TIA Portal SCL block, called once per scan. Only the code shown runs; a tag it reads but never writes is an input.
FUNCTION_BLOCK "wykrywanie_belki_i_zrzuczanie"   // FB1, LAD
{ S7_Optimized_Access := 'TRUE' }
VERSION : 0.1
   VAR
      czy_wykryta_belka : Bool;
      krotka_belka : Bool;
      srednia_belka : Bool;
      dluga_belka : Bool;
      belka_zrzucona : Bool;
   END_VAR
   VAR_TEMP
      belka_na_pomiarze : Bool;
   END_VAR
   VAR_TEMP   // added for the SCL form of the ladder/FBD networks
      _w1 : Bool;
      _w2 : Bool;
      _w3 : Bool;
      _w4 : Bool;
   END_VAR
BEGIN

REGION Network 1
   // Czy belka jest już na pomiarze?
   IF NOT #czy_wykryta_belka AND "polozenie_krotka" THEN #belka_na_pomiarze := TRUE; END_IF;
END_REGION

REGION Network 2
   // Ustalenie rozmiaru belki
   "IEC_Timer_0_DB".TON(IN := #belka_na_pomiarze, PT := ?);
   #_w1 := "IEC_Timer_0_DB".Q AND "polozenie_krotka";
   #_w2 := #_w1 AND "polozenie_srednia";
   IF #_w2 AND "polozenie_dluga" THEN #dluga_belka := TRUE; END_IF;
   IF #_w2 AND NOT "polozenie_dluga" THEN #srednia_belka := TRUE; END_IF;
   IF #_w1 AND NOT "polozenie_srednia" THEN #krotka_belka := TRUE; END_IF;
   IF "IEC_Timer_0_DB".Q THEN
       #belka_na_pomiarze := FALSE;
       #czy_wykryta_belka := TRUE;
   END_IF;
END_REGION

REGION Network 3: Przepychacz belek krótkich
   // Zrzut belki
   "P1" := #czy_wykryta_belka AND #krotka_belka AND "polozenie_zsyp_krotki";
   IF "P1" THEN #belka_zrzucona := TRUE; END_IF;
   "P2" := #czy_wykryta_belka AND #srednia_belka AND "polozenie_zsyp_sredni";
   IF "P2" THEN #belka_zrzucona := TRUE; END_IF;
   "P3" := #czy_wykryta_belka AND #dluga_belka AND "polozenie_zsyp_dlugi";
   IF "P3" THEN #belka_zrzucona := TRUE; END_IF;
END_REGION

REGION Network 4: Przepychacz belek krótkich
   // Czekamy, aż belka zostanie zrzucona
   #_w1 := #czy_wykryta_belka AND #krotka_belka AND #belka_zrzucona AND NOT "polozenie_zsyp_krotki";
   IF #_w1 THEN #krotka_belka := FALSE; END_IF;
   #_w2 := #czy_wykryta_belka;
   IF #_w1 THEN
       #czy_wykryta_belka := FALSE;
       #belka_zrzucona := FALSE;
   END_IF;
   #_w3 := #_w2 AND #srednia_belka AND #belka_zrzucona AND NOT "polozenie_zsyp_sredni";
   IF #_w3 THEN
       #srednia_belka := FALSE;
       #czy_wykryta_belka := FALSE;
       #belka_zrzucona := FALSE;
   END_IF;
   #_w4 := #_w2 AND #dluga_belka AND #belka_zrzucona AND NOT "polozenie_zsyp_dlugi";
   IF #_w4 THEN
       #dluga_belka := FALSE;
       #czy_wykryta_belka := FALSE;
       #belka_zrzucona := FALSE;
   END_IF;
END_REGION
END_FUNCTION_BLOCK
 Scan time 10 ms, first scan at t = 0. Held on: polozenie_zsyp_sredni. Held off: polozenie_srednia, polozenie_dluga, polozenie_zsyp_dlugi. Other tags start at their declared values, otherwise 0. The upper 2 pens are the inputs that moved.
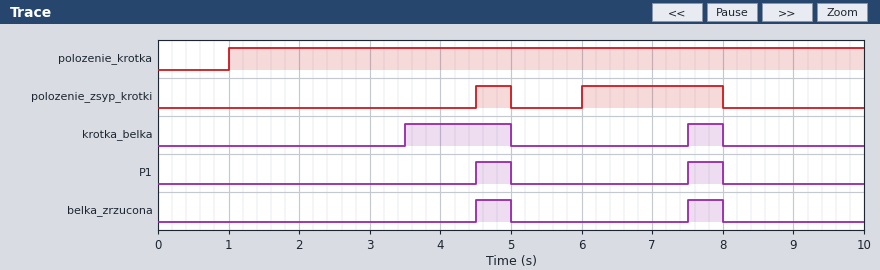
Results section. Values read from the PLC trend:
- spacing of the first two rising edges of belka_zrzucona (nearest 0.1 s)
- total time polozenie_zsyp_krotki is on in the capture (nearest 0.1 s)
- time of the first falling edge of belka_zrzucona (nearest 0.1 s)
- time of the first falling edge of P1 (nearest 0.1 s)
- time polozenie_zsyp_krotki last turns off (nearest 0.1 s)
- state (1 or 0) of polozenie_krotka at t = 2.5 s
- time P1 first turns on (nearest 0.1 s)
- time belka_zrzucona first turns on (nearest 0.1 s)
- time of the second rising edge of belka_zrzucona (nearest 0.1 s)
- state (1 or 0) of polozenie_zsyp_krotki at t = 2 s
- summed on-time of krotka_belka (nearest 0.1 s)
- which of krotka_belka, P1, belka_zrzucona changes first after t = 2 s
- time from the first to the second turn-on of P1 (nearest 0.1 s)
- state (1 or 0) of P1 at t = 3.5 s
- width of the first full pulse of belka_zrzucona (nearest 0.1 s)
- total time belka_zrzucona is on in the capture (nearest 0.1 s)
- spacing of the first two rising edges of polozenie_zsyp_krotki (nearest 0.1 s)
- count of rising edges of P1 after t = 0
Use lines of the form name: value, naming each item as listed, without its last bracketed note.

spacing of the first two rising edges of belka_zrzucona: 3.0 s
total time polozenie_zsyp_krotki is on in the capture: 2.5 s
time of the first falling edge of belka_zrzucona: 5.0 s
time of the first falling edge of P1: 5.0 s
time polozenie_zsyp_krotki last turns off: 8.0 s
state (1 or 0) of polozenie_krotka at t = 2.5 s: 1
time P1 first turns on: 4.5 s
time belka_zrzucona first turns on: 4.5 s
time of the second rising edge of belka_zrzucona: 7.5 s
state (1 or 0) of polozenie_zsyp_krotki at t = 2 s: 0
summed on-time of krotka_belka: 2.0 s
which of krotka_belka, P1, belka_zrzucona changes first after t = 2 s: krotka_belka
time from the first to the second turn-on of P1: 3.0 s
state (1 or 0) of P1 at t = 3.5 s: 0
width of the first full pulse of belka_zrzucona: 0.5 s
total time belka_zrzucona is on in the capture: 1.0 s
spacing of the first two rising edges of polozenie_zsyp_krotki: 1.5 s
count of rising edges of P1 after t = 0: 2
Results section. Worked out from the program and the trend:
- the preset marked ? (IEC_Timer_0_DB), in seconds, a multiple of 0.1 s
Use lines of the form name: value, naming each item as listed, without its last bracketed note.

the preset marked ? (IEC_Timer_0_DB), in seconds, a multiple of 0.1 s: 2.5 s
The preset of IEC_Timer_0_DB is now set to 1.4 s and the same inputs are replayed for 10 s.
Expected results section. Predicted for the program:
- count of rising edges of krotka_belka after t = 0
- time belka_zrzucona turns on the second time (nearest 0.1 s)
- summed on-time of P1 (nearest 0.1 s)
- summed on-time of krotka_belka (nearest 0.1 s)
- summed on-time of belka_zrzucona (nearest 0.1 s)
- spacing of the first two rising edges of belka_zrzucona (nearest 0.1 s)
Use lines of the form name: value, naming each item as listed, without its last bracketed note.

count of rising edges of krotka_belka after t = 0: 3
time belka_zrzucona turns on the second time: 6.4 s
summed on-time of P1: 2.1 s
summed on-time of krotka_belka: 4.8 s
summed on-time of belka_zrzucona: 2.1 s
spacing of the first two rising edges of belka_zrzucona: 1.9 s
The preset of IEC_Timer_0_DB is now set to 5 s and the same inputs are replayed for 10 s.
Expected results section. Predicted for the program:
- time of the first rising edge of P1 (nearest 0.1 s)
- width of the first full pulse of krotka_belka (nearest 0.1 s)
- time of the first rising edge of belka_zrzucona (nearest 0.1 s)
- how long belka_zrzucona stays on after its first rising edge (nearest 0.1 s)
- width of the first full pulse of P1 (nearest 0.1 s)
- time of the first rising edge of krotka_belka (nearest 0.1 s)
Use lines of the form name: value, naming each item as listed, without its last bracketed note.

time of the first rising edge of P1: 6.0 s
width of the first full pulse of krotka_belka: 2.0 s
time of the first rising edge of belka_zrzucona: 6.0 s
how long belka_zrzucona stays on after its first rising edge: 2.0 s
width of the first full pulse of P1: 2.0 s
time of the first rising edge of krotka_belka: 6.0 s
